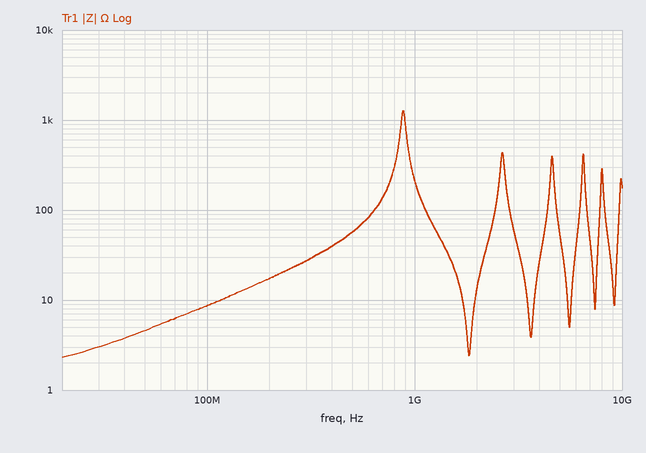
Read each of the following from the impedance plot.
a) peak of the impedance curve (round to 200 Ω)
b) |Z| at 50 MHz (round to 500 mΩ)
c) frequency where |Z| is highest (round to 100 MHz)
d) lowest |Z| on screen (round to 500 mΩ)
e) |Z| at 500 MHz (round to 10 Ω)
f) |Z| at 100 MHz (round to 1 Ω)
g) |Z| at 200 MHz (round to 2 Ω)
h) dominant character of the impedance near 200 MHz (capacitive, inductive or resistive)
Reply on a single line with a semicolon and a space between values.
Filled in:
1.2 kΩ; 4.5 Ω; 900 MHz; 2.5 Ω; 60 Ω; 9 Ω; 18 Ω; inductive
